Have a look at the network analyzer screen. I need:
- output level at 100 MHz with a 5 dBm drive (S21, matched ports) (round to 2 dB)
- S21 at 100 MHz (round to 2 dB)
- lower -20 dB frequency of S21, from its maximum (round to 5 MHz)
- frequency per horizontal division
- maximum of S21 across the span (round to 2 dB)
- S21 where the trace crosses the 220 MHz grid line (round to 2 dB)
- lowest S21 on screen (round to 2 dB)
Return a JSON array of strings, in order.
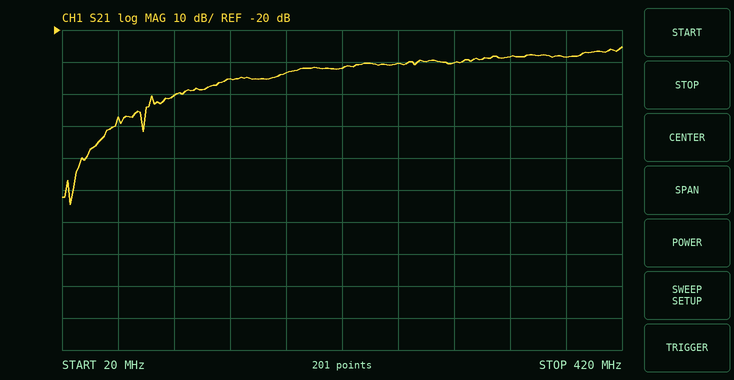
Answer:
["-36 dBm", "-40 dB", "80 MHz", "40 MHz", "-26 dB", "-32 dB", "-74 dB"]
